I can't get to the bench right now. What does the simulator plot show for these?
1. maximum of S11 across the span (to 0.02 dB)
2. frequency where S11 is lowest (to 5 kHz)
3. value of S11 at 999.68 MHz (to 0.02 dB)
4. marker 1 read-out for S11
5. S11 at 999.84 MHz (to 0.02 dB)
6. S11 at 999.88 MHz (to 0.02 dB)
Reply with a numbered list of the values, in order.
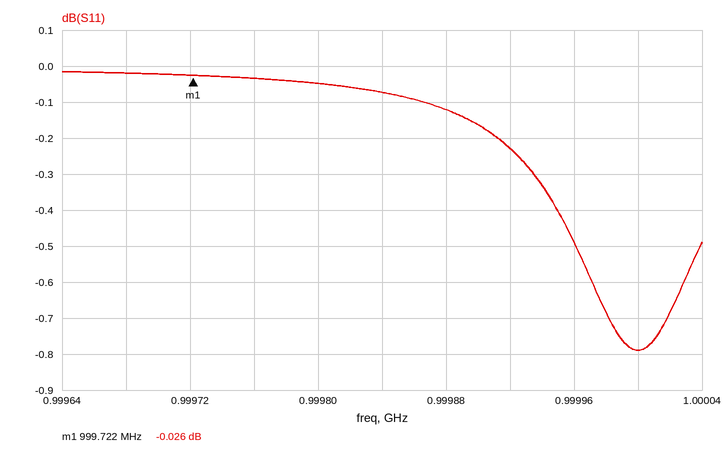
1. -0.02 dB
2. 1.000000 GHz
3. -0.02 dB
4. -0.026 dB
5. -0.08 dB
6. -0.12 dB
